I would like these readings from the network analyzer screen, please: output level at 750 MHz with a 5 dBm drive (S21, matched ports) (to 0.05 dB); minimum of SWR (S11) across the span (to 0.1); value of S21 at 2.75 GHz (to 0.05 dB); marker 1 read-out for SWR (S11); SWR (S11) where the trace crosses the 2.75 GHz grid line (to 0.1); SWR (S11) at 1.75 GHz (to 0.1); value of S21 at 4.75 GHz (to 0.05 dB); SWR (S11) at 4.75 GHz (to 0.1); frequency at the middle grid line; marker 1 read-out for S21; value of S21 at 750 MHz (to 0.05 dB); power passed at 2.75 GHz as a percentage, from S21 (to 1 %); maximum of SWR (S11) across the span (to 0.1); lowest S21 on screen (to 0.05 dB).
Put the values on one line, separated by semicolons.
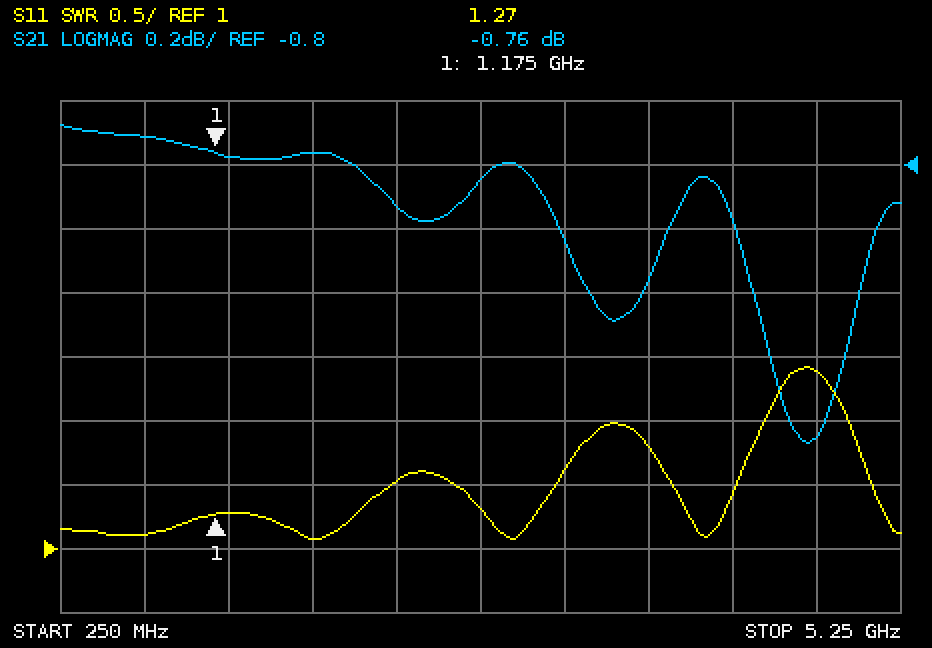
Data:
4.30 dBm; 1.1; -0.85 dB; 1.27; 1.3; 1.1; -1.65 dB; 2.4; 2.75 GHz; -0.76 dB; -0.70 dB; 82 %; 2.4; -1.65 dB
